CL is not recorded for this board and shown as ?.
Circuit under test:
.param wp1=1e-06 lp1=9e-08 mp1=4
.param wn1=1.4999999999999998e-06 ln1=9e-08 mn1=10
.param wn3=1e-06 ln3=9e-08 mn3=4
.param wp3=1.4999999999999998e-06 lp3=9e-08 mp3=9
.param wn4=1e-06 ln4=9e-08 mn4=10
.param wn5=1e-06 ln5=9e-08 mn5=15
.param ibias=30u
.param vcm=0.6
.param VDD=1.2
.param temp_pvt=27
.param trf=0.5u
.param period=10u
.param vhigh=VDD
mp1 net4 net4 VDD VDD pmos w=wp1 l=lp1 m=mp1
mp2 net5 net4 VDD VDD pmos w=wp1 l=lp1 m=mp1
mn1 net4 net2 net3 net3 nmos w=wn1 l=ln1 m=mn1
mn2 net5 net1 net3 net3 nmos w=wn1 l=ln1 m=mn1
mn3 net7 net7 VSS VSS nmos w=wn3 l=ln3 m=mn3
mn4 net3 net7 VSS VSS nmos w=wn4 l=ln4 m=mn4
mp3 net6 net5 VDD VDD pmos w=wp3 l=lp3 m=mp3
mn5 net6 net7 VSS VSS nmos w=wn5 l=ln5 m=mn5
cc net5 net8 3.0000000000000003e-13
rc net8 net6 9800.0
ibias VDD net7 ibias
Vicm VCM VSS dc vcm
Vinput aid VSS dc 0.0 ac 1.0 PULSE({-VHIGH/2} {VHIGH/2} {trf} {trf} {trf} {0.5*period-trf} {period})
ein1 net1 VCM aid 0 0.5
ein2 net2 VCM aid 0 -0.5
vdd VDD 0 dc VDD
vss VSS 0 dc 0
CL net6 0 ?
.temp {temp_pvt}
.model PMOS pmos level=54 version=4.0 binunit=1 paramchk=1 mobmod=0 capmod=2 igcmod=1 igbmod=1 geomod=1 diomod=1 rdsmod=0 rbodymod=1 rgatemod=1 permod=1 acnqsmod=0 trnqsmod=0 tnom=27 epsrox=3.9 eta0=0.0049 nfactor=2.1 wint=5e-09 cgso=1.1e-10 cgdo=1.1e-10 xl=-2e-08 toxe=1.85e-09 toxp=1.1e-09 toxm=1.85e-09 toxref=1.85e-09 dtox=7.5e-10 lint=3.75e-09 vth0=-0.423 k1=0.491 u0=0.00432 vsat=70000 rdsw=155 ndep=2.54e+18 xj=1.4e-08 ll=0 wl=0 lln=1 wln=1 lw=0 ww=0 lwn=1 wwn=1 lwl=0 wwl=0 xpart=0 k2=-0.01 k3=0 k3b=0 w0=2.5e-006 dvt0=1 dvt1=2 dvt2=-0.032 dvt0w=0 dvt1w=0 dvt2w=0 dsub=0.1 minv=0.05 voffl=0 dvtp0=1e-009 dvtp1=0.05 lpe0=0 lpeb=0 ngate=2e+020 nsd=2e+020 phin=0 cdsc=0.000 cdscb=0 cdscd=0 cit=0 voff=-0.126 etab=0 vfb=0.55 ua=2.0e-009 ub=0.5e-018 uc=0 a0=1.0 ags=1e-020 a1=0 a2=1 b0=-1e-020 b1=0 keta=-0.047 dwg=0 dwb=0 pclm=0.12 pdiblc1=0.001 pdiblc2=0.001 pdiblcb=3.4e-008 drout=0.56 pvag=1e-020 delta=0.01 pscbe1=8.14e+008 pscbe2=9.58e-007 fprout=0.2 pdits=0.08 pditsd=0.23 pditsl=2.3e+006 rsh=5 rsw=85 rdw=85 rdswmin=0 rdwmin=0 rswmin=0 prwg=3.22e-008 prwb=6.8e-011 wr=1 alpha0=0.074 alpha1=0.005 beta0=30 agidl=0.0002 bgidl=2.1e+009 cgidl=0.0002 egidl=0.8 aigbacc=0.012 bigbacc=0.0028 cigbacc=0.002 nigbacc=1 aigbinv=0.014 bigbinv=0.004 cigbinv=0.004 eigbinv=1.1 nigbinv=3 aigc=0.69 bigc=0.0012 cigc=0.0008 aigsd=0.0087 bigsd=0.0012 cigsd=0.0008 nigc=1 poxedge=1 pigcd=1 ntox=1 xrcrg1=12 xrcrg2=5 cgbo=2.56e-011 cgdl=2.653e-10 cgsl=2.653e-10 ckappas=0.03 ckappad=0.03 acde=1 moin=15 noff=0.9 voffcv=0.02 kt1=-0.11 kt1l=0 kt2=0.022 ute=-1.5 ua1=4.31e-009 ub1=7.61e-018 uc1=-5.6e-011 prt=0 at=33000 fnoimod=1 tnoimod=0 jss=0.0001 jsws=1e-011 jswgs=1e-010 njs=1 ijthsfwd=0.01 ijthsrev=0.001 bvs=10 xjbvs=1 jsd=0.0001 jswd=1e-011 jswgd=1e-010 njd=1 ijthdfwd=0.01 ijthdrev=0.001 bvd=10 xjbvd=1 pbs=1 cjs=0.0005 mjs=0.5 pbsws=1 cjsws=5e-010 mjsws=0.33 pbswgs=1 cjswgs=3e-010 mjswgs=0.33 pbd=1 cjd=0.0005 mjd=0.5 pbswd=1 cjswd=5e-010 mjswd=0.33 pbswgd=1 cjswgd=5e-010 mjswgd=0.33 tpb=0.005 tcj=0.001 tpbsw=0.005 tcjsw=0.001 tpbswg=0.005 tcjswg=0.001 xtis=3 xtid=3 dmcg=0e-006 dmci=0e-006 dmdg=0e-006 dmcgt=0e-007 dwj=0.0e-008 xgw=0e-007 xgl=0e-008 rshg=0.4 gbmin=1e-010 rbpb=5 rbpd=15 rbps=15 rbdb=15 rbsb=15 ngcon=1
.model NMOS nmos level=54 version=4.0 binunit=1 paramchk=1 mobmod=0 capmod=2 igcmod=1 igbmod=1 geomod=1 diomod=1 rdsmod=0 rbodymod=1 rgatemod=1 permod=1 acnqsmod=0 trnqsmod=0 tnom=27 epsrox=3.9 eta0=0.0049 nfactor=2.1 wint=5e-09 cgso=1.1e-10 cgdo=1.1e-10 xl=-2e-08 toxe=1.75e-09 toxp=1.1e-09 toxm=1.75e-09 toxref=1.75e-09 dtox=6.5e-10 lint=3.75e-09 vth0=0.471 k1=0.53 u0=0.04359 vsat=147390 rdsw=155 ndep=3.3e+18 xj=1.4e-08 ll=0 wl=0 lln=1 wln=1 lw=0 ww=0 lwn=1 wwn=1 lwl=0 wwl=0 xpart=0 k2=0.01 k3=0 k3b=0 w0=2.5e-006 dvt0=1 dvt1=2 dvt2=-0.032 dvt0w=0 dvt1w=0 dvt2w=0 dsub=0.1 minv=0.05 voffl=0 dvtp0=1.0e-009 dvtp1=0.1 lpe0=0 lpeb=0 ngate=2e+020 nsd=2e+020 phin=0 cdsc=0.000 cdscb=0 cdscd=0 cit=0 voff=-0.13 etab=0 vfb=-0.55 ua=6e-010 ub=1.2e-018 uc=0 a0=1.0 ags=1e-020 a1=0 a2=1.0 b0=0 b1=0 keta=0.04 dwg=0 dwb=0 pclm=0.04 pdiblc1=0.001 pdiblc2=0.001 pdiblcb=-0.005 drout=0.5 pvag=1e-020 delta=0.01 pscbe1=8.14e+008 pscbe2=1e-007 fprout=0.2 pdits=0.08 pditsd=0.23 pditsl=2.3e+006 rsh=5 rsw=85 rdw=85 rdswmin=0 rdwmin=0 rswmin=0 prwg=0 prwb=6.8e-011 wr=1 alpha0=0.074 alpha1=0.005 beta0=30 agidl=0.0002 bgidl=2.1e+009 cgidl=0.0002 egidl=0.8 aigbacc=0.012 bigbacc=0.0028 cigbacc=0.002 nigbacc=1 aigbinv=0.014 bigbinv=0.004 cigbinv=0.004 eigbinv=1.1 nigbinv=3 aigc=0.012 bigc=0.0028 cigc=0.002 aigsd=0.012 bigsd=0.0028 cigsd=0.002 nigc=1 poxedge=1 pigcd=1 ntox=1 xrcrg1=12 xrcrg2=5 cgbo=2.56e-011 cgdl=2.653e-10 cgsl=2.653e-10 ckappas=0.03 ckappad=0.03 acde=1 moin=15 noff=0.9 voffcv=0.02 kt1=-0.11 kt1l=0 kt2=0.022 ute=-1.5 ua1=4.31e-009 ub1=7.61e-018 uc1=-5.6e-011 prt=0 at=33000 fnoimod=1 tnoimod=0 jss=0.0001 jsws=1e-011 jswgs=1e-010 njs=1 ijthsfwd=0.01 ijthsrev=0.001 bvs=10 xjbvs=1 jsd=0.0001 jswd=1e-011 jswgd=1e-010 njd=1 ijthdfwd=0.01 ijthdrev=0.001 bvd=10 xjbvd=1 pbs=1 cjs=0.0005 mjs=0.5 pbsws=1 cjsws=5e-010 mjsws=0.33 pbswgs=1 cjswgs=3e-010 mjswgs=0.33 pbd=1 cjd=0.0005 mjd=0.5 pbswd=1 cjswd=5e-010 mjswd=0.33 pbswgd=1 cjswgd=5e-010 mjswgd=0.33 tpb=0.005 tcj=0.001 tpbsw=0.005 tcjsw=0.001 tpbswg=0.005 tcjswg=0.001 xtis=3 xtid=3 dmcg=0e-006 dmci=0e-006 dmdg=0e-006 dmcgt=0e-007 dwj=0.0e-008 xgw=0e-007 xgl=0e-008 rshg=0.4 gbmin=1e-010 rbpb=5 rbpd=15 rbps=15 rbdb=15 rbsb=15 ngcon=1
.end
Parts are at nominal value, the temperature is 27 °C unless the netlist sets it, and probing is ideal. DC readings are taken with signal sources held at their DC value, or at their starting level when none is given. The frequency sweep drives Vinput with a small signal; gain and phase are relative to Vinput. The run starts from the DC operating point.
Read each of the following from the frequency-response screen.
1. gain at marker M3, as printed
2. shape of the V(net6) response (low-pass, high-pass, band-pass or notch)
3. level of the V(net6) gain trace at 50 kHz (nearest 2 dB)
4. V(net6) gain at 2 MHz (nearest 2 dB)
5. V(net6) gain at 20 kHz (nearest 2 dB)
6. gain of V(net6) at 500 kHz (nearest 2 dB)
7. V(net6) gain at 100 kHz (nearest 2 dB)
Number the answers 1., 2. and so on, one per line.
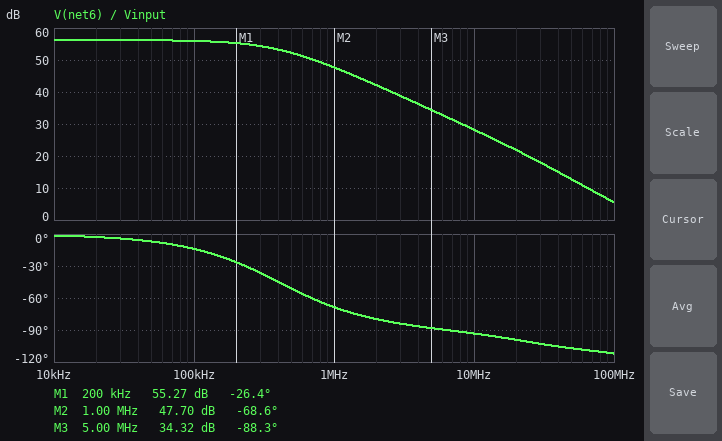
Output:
1. 34.32 dB
2. low-pass
3. 56 dB
4. 42 dB
5. 56 dB
6. 52 dB
7. 56 dB
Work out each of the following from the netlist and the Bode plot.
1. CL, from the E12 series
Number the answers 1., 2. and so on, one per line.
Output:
1. 5.6 pF
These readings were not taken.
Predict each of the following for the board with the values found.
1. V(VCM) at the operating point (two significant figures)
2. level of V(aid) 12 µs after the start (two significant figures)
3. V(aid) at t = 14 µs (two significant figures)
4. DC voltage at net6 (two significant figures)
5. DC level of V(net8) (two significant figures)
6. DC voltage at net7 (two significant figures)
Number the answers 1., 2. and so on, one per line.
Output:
1. 600 mV
2. 600 mV
3. 600 mV
4. 620 mV
5. 620 mV
6. 430 mV
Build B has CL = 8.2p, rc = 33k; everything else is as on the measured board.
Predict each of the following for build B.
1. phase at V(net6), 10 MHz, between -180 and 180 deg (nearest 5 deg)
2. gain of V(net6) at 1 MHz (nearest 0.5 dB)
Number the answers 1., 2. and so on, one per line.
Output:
1. -85 deg
2. 47.0 dB
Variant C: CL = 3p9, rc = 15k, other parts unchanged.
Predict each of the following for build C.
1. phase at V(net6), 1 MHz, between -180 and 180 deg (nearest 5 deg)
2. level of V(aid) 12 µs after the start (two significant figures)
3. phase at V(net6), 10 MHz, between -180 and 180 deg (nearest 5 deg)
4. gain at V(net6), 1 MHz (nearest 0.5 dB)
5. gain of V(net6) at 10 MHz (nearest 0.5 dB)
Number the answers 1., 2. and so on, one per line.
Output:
1. -65 deg
2. 600 mV
3. -85 deg
4. 48.0 dB
5. 29.0 dB
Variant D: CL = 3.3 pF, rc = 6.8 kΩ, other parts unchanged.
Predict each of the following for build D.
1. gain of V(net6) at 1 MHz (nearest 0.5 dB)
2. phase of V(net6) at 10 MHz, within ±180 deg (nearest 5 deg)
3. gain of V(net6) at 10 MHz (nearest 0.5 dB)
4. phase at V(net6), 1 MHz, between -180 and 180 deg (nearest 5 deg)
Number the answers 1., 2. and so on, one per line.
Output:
1. 48.5 dB
2. -90 deg
3. 29.0 dB
4. -65 deg
